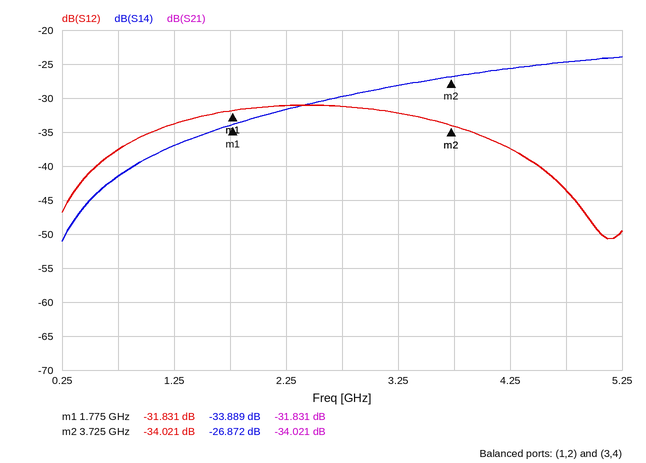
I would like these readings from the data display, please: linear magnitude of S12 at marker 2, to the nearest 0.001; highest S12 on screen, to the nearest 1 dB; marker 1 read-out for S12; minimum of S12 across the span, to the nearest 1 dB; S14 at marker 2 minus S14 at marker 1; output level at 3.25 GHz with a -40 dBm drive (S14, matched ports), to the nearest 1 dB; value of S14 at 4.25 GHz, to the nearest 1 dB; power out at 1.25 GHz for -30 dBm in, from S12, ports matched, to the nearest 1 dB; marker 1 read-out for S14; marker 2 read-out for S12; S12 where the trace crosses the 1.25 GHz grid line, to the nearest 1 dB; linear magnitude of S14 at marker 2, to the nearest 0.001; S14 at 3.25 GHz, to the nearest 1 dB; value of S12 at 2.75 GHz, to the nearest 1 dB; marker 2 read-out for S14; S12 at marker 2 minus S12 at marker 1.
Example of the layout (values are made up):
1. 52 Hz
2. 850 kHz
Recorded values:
1. 0.020
2. -31 dB
3. -31.831 dB
4. -51 dB
5. 7.017 dB
6. -68 dBm
7. -26 dB
8. -64 dBm
9. -33.889 dB
10. -34.021 dB
11. -34 dB
12. 0.045
13. -28 dB
14. -31 dB
15. -26.872 dB
16. -2.190 dB
